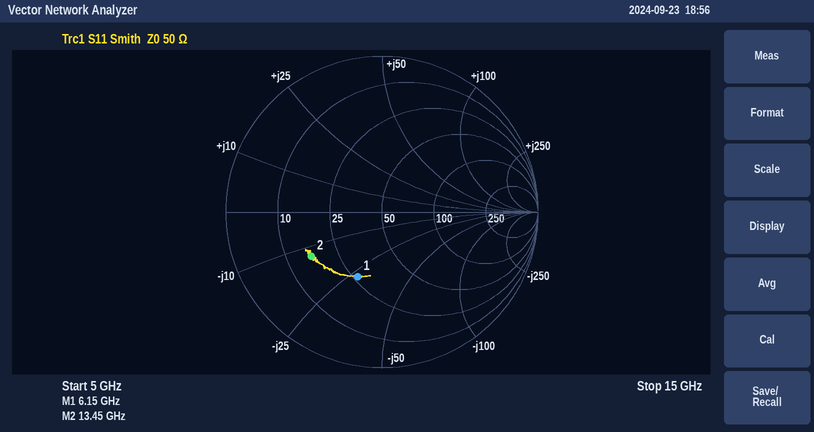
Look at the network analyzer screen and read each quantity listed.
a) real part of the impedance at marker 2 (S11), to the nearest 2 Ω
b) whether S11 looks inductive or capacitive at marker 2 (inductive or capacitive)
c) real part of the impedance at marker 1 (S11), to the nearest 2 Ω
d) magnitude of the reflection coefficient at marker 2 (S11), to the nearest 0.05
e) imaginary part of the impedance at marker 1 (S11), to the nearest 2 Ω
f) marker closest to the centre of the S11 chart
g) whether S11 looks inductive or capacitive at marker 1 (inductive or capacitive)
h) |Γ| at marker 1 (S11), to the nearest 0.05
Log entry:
16 Ω
capacitive
26 Ω
0.55
-28 Ω
marker 1
capacitive
0.45
